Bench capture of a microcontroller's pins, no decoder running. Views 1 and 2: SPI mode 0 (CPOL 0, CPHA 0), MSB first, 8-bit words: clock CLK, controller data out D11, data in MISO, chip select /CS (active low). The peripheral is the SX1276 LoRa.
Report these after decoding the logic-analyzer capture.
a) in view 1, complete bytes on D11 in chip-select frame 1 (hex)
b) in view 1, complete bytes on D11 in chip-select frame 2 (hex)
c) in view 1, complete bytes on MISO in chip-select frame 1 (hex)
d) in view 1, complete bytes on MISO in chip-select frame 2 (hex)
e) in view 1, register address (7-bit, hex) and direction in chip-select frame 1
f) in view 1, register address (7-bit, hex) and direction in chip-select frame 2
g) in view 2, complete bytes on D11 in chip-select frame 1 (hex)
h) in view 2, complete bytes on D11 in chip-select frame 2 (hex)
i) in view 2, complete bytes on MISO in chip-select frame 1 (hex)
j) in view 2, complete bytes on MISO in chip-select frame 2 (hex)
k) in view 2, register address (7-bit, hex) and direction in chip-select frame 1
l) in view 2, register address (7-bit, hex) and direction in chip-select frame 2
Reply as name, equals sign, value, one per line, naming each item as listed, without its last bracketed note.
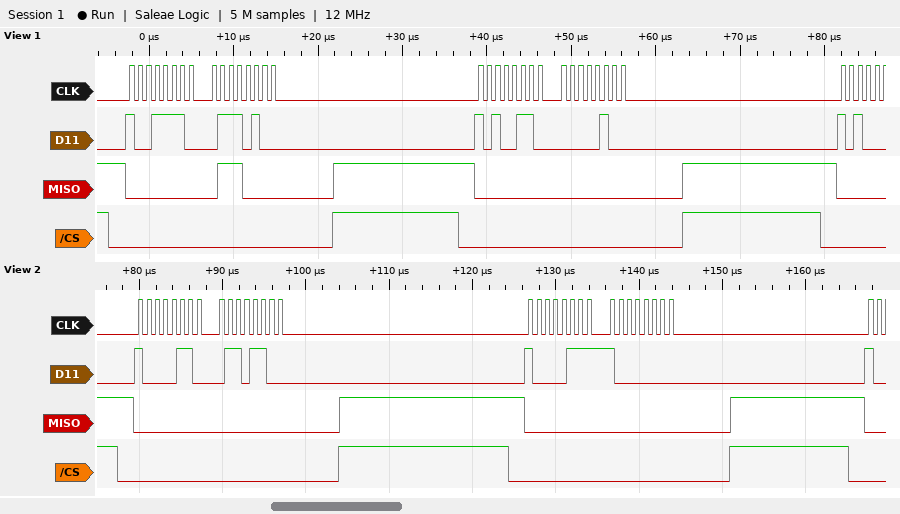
in view 1, complete bytes on D11 in chip-select frame 1 = 0x9E 0x74
in view 1, complete bytes on D11 in chip-select frame 2 = 0xA6 0x04
in view 1, complete bytes on MISO in chip-select frame 1 = 0x00 0x70
in view 1, complete bytes on MISO in chip-select frame 2 = 0x00 0x00
in view 1, register address (7-bit, hex) and direction in chip-select frame 1 = 0x1E write
in view 1, register address (7-bit, hex) and direction in chip-select frame 2 = 0x26 write
in view 2, complete bytes on D11 in chip-select frame 1 = 86 6C
in view 2, complete bytes on D11 in chip-select frame 2 = 87 80
in view 2, complete bytes on MISO in chip-select frame 1 = 00 00
in view 2, complete bytes on MISO in chip-select frame 2 = 00 00
in view 2, register address (7-bit, hex) and direction in chip-select frame 1 = 0x06 write
in view 2, register address (7-bit, hex) and direction in chip-select frame 2 = 0x07 write
